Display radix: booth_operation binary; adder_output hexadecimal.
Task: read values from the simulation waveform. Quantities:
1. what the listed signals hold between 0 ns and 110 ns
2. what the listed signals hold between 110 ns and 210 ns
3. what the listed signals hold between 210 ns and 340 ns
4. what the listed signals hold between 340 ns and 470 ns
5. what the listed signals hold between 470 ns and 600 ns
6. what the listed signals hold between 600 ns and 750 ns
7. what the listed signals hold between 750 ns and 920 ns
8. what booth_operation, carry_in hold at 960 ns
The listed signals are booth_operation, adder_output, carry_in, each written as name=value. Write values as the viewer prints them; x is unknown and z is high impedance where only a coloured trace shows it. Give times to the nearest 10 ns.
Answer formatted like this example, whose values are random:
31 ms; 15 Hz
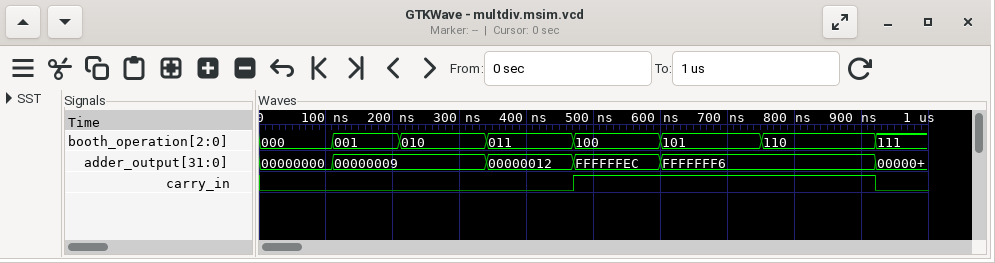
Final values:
booth_operation=000, adder_output=00000000, carry_in=0; booth_operation=001, adder_output=00000009, carry_in=0; booth_operation=010, adder_output=00000009, carry_in=0; booth_operation=011, adder_output=00000012, carry_in=0; booth_operation=100, adder_output=FFFFFFEC, carry_in=1; booth_operation=101, adder_output=FFFFFFF6, carry_in=1; booth_operation=110, adder_output=FFFFFFF6, carry_in=1; booth_operation=111, carry_in=0
